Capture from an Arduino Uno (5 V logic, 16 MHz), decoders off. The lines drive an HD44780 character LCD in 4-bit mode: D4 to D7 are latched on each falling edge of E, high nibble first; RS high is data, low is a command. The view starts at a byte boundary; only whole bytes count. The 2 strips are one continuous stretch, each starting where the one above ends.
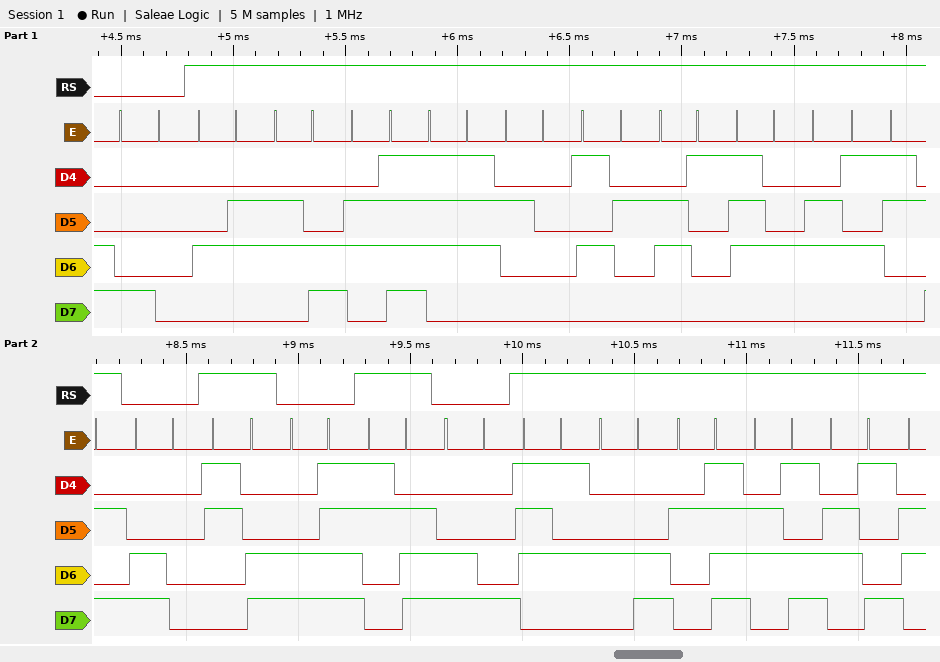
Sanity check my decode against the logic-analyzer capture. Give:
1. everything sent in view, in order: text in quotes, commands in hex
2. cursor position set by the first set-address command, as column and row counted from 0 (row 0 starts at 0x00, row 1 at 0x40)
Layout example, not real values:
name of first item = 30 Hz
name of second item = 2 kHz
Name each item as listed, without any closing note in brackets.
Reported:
everything sent in view, in order: text in quotes, commands in hex = 0x80 "Flow Rate:" 0xC0 "<" 0xCF ">" 0xC8 "uL/mi"
cursor position set by the first set-address command, as column and row counted from 0 = column 0, row 0
